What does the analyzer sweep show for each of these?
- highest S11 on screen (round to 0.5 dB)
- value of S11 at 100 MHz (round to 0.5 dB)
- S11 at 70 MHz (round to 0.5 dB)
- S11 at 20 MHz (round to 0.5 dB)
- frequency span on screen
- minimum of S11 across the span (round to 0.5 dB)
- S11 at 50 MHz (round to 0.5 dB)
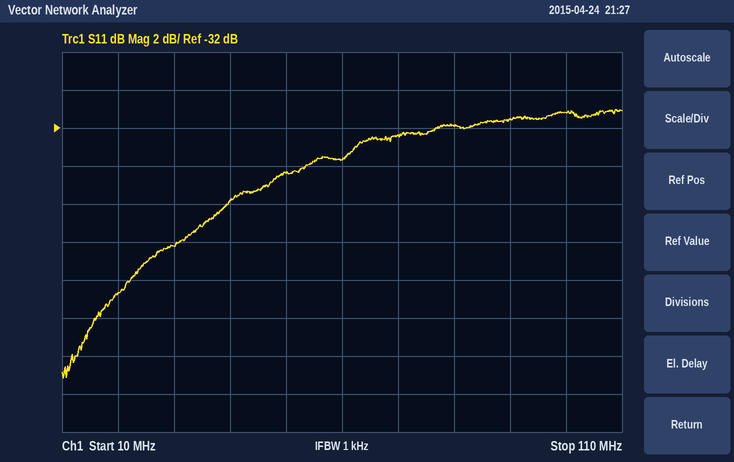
-31.0 dB
-31.0 dB
-32.5 dB
-40.5 dB
100 MHz
-45.0 dB
-34.5 dB
